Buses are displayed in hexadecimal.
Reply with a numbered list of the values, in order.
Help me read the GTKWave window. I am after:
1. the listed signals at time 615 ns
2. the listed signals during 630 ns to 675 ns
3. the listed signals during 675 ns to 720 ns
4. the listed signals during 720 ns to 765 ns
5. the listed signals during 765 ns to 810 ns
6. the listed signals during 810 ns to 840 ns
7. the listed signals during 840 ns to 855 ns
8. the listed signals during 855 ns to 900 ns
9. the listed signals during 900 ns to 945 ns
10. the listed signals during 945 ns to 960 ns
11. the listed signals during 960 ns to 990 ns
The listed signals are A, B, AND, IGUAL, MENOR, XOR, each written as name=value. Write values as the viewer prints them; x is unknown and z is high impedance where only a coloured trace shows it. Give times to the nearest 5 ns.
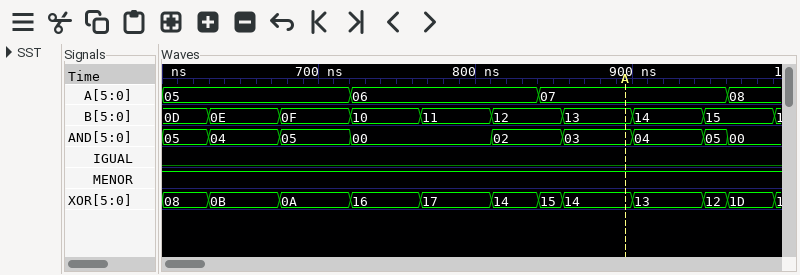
1. A=05, B=0D, AND=05, IGUAL=0, MENOR=1, XOR=08
2. A=05, B=0E, AND=04, IGUAL=0, MENOR=1, XOR=0B
3. A=05, B=0F, AND=05, IGUAL=0, MENOR=1, XOR=0A
4. A=06, B=10, AND=00, IGUAL=0, MENOR=1, XOR=16
5. A=06, B=11, AND=00, IGUAL=0, MENOR=1, XOR=17
6. A=06, B=12, AND=02, IGUAL=0, MENOR=1, XOR=14
7. A=07, B=12, AND=02, IGUAL=0, MENOR=1, XOR=15
8. A=07, B=13, AND=03, IGUAL=0, MENOR=1, XOR=14
9. A=07, B=14, AND=04, IGUAL=0, MENOR=1, XOR=13
10. A=07, B=15, AND=05, IGUAL=0, MENOR=1, XOR=12
11. A=08, B=15, AND=00, IGUAL=0, MENOR=1, XOR=1D
